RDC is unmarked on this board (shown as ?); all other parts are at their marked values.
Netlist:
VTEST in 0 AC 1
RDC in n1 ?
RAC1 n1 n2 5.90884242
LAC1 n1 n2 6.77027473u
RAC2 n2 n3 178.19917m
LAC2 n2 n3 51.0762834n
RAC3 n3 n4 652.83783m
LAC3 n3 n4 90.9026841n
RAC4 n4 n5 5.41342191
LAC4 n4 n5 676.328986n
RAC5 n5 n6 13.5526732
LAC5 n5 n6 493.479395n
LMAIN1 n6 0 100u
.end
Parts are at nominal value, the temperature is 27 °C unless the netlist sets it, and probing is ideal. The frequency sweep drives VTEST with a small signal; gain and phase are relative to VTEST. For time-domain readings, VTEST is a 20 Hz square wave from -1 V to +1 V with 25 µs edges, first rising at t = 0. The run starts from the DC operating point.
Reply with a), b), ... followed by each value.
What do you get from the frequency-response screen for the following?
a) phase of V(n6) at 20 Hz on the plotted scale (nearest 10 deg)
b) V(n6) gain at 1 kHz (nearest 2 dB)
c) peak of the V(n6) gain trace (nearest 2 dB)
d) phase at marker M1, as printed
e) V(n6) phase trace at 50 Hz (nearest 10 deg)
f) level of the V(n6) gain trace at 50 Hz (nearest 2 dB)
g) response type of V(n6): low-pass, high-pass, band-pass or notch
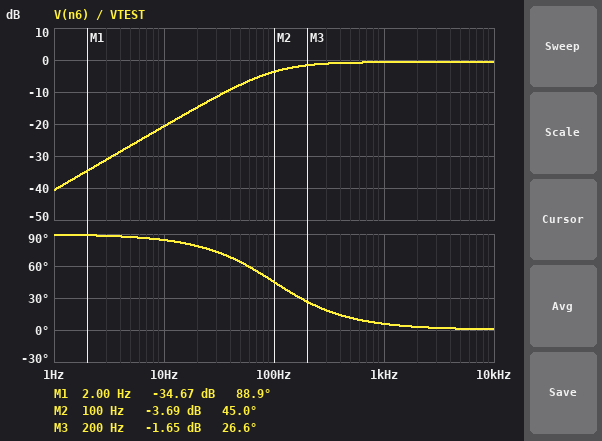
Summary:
a) 80 deg
b) 0 dB
c) 0 dB
d) 88.9 deg
e) 60 deg
f) -8 dB
g) high-pass
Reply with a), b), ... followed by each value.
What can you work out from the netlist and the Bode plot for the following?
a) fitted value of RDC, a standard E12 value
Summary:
a) 0.068 Ω
